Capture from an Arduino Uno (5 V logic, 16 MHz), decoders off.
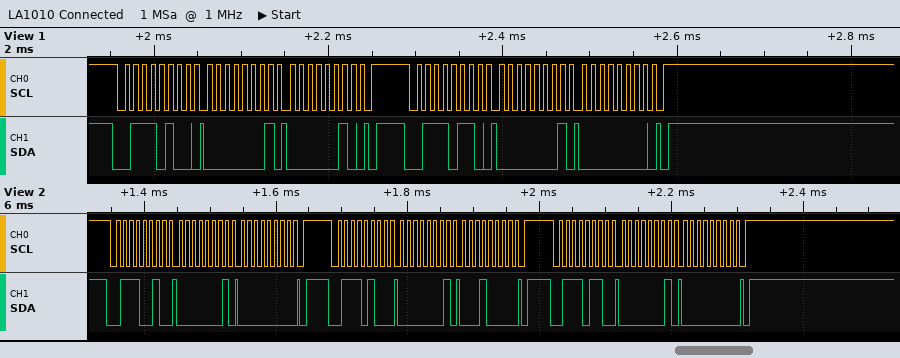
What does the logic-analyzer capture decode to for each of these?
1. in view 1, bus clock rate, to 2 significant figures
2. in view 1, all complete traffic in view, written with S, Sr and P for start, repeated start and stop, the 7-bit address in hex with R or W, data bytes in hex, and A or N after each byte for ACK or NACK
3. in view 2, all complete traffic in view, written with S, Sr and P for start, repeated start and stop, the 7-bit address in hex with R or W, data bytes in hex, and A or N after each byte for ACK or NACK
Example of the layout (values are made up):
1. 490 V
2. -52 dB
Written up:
1. 100 kHz
2. S 3AW A 01 A 02 A P S 3BW A 01 A 00 A P
3. S 39W A 01 A 00 A P S 3AW A 01 A 10 A P S 3BW A 01 A 00 A P
